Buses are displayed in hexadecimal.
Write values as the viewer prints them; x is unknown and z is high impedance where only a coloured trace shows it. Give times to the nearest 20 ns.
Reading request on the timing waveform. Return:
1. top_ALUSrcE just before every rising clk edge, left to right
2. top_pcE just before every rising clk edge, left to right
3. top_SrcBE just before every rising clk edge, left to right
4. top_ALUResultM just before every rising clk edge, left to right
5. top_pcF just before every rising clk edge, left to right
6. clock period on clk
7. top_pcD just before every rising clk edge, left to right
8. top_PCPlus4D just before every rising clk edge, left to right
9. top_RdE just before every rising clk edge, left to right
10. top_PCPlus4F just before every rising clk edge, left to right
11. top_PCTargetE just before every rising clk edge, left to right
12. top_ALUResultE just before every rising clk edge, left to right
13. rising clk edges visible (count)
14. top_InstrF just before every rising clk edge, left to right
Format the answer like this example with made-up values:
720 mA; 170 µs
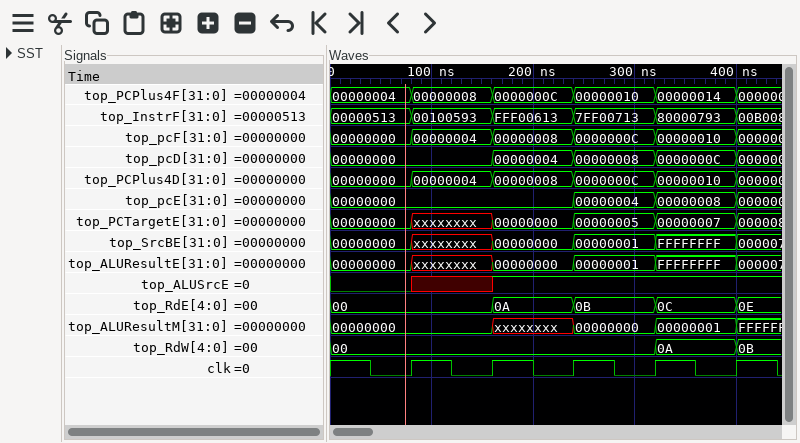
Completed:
0 x 1 1 1; 00000000, 00000000, 00000000, 00000004, 00000008; 00000000, xxxxxxxx, 00000000, 00000001, FFFFFFFF; 00000000, 00000000, xxxxxxxx, 00000000, 00000001; 00000000, 00000004, 00000008, 0000000C, 00000010; 80 ns; 00000000, 00000000, 00000004, 00000008, 0000000C; 00000000, 00000004, 00000008, 0000000C, 00000010; 00, 00, 0A, 0B, 0C; 00000004, 00000008, 0000000C, 00000010, 00000014; 00000000, xxxxxxxx, 00000000, 00000005, 00000007; 00000000, xxxxxxxx, 00000000, 00000001, FFFFFFFF; 5; 00000513, 00100593, FFF00613, 7FF00713, 80000793
